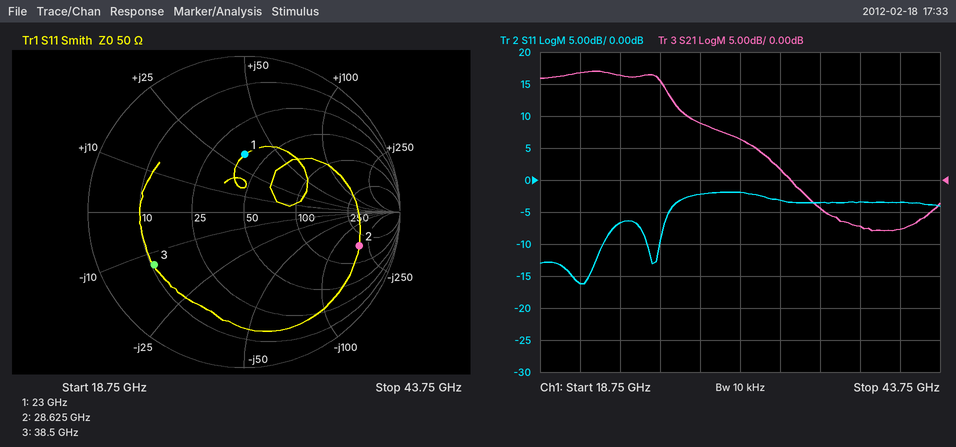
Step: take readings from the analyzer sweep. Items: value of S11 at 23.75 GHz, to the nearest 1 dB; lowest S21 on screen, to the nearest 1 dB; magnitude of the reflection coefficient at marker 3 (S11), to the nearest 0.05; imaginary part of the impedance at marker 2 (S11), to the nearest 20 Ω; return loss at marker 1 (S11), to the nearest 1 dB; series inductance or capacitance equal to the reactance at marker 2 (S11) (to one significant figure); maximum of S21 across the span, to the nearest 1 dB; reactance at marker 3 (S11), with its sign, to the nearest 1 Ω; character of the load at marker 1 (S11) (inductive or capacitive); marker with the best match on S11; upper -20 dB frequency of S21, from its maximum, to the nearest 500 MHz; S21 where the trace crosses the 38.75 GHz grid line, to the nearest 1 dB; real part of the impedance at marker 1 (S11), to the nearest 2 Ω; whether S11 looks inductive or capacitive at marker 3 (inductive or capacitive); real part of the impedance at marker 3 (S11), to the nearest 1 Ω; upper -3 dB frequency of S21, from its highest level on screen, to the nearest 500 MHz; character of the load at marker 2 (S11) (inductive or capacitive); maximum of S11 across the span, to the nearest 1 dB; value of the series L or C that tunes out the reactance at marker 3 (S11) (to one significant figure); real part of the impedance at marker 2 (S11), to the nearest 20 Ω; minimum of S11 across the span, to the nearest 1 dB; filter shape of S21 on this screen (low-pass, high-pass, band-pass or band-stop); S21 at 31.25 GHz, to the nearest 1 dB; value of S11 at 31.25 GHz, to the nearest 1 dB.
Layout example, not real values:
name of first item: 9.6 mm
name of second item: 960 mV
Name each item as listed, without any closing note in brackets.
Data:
value of S11 at 23.75 GHz, to the nearest 1 dB: -7 dB
lowest S21 on screen, to the nearest 1 dB: -8 dB
magnitude of the reflection coefficient at marker 3 (S11), to the nearest 0.05: 0.65
imaginary part of the impedance at marker 2 (S11), to the nearest 20 Ω: -180 Ω
return loss at marker 1 (S11), to the nearest 1 dB: 9 dB
series inductance or capacitance equal to the reactance at marker 2 (S11): 30 fF
maximum of S21 across the span, to the nearest 1 dB: 17 dB
reactance at marker 3 (S11), with its sign, to the nearest 1 Ω: -13 Ω
character of the load at marker 1 (S11): inductive
marker with the best match on S11: marker 1
upper -20 dB frequency of S21, from its maximum, to the nearest 500 MHz: 35.5 GHz
S21 where the trace crosses the 38.75 GHz grid line, to the nearest 1 dB: -7 dB
real part of the impedance at marker 1 (S11), to the nearest 2 Ω: 38 Ω
whether S11 looks inductive or capacitive at marker 3: capacitive
real part of the impedance at marker 3 (S11), to the nearest 1 Ω: 11 Ω
upper -3 dB frequency of S21, from its highest level on screen, to the nearest 500 MHz: 26.5 GHz
character of the load at marker 2 (S11): capacitive
maximum of S11 across the span, to the nearest 1 dB: -2 dB
value of the series L or C that tunes out the reactance at marker 3 (S11): 50 pH
real part of the impedance at marker 2 (S11), to the nearest 20 Ω: 180 Ω
minimum of S11 across the span, to the nearest 1 dB: -16 dB
filter shape of S21 on this screen: low-pass
S21 at 31.25 GHz, to the nearest 1 dB: 6 dB
value of S11 at 31.25 GHz, to the nearest 1 dB: -2 dB
